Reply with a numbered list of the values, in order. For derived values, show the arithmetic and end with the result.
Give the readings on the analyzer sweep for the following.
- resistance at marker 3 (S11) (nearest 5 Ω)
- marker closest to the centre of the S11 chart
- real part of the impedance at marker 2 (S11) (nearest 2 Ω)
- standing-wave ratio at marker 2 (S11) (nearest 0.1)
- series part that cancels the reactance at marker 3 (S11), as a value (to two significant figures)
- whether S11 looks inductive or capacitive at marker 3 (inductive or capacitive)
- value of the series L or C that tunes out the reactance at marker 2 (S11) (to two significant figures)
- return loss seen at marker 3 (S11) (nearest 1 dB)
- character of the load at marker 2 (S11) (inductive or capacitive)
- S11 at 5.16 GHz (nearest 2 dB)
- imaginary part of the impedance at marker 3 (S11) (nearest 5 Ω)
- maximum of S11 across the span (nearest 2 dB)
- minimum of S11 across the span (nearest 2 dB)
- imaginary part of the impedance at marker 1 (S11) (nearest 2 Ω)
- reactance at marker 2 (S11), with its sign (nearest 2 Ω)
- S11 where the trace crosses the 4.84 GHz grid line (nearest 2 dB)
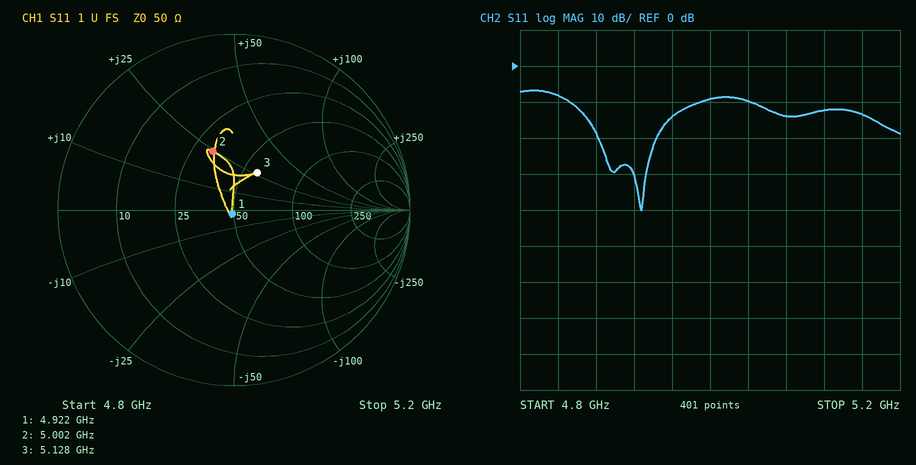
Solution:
1. 60 Ω
2. marker 1
3. 32 Ω
4. 2.1
5. C = 1/(2π × 5.128 GHz × 25 Ω) ≈ 1.2 pF
6. inductive
7. C = 1/(2π × 5.002 GHz × 24 Ω) ≈ 1.3 pF
8. 12 dB
9. inductive
10. -14 dB
11. +25 Ω
12. -6 dB
13. -40 dB
14. -2 Ω
15. +24 Ω
16. -8 dB
